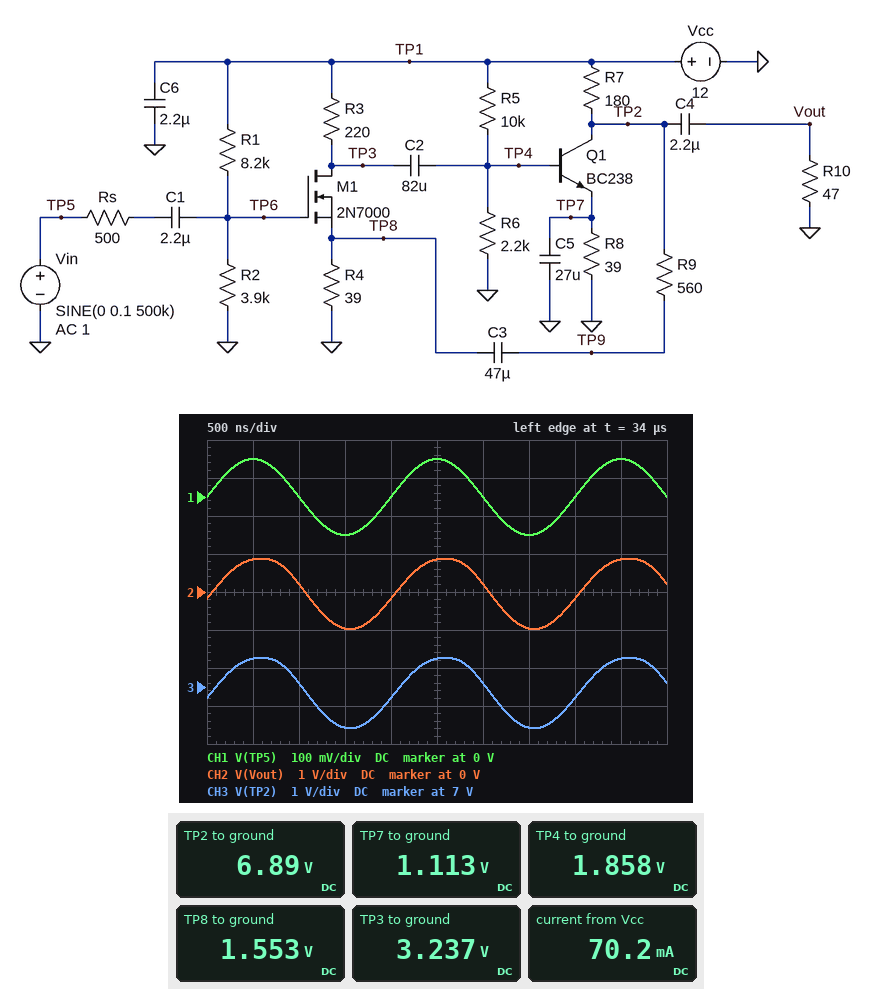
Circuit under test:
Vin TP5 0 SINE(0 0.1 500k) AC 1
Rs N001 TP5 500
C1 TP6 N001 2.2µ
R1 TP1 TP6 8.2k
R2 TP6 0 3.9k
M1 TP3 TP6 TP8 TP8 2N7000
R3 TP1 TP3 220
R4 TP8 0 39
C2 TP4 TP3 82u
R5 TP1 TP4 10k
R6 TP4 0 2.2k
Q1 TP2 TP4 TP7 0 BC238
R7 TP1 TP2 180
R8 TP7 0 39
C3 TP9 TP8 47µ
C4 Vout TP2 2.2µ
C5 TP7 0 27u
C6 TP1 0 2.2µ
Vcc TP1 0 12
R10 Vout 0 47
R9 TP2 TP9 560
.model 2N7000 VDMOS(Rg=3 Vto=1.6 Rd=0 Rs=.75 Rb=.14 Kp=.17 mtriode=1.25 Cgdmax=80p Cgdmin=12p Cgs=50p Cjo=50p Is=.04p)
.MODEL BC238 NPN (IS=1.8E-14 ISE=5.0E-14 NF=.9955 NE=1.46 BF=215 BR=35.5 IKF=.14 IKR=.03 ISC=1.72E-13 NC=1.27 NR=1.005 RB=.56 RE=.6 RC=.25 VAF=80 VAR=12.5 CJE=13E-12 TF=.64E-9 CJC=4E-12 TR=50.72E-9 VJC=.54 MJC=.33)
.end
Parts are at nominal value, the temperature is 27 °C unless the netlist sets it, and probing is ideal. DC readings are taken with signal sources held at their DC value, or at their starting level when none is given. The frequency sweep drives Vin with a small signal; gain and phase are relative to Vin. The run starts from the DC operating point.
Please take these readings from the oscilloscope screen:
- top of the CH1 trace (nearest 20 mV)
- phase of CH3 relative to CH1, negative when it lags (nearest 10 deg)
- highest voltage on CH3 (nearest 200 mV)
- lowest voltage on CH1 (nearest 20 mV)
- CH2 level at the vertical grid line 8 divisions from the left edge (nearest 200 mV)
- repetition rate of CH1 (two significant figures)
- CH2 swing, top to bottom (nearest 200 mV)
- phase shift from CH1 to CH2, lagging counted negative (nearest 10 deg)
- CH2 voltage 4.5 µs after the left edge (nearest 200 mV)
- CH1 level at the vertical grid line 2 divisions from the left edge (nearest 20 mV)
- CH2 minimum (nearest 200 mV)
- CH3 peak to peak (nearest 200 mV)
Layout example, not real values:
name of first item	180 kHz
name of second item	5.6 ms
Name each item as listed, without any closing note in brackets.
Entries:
top of the CH1 trace	100 mV
phase of CH3 relative to CH1, negative when it lags	-10 deg
highest voltage on CH3	7.8 V
lowest voltage on CH1	-100 mV
CH2 level at the vertical grid line 8 divisions from the left edge	-200 mV
repetition rate of CH1	500 kHz
CH2 swing, top to bottom	1.8 V
phase shift from CH1 to CH2, lagging counted negative	-10 deg
CH2 voltage 4.5 µs after the left edge	800 mV
CH1 level at the vertical grid line 2 divisions from the left edge	0 V
CH2 minimum	-1.0 V
CH3 peak to peak	1.8 V
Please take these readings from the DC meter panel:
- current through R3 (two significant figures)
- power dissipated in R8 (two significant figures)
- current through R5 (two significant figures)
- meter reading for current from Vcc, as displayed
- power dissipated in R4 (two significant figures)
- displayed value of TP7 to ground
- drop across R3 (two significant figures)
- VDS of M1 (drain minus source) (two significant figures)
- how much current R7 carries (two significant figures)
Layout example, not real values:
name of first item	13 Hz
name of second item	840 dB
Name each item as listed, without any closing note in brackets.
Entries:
current through R3	40 mA
power dissipated in R8	32 mW
current through R5	1.0 mA
meter reading for current from Vcc, as displayed	70.2 mA
power dissipated in R4	62 mW
displayed value of TP7 to ground	1.113 V
drop across R3	8.8 V
VDS of M1 (drain minus source)	1.7 V
how much current R7 carries	28 mA
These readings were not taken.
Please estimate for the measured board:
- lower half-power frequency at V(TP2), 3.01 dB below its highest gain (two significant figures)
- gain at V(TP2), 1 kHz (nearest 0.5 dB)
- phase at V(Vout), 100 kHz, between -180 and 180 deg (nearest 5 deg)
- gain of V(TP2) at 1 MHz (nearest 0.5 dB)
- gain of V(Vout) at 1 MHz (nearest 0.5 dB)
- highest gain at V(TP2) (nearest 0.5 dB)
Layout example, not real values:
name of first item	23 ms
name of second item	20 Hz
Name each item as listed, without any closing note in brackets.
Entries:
lower half-power frequency at V(TP2), 3.01 dB below its highest gain	130 Hz
gain at V(TP2), 1 kHz	19.5 dB
phase at V(Vout), 100 kHz, between -180 and 180 deg	0 deg
gain of V(TP2) at 1 MHz	19.5 dB
gain of V(Vout) at 1 MHz	19.5 dB
highest gain at V(TP2)	20.0 dB
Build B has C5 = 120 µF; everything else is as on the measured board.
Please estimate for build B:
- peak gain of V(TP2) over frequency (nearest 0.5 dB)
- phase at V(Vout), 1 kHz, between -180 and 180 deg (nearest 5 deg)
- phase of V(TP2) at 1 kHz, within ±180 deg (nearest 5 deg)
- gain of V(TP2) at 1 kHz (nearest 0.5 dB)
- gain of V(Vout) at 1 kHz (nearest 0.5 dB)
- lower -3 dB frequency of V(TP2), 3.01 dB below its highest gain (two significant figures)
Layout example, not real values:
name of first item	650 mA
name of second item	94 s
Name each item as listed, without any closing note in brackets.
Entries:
peak gain of V(TP2) over frequency	21.0 dB
phase at V(Vout), 1 kHz, between -180 and 180 deg	55 deg
phase of V(TP2) at 1 kHz, within ±180 deg	0 deg
gain of V(TP2) at 1 kHz	20.5 dB
gain of V(Vout) at 1 kHz	15.5 dB
lower -3 dB frequency of V(TP2), 3.01 dB below its highest gain	48 Hz
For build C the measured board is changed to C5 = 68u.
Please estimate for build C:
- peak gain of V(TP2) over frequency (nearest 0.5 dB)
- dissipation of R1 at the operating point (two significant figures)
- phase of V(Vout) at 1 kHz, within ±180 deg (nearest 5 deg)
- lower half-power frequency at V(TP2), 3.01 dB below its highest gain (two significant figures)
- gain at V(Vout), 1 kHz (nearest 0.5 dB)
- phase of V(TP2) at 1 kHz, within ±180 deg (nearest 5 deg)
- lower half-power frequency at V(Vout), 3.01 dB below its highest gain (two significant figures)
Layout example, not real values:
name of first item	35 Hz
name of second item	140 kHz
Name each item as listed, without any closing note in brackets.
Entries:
peak gain of V(TP2) over frequency	20.5 dB
dissipation of R1 at the operating point	8.1 mW
phase of V(Vout) at 1 kHz, within ±180 deg	60 deg
lower half-power frequency at V(TP2), 3.01 dB below its highest gain	66 Hz
gain at V(Vout), 1 kHz	15.0 dB
phase of V(TP2) at 1 kHz, within ±180 deg	0 deg
lower half-power frequency at V(Vout), 3.01 dB below its highest gain	1.4 kHz
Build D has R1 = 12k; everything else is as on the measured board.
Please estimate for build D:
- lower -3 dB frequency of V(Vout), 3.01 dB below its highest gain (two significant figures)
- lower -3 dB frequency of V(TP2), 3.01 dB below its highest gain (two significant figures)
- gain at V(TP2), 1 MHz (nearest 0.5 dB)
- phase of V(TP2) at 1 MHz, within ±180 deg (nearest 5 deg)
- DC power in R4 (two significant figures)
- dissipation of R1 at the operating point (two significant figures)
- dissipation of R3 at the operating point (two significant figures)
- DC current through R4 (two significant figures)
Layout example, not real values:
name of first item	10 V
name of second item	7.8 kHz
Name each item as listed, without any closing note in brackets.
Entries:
lower -3 dB frequency of V(Vout), 3.01 dB below its highest gain	1.7 kHz
lower -3 dB frequency of V(TP2), 3.01 dB below its highest gain	140 Hz
gain at V(TP2), 1 MHz	20.0 dB
phase of V(TP2) at 1 MHz, within ±180 deg	-10 deg
DC power in R4	18 mW
dissipation of R1 at the operating point	6.8 mW
dissipation of R3 at the operating point	99 mW
DC current through R4	21 mA
